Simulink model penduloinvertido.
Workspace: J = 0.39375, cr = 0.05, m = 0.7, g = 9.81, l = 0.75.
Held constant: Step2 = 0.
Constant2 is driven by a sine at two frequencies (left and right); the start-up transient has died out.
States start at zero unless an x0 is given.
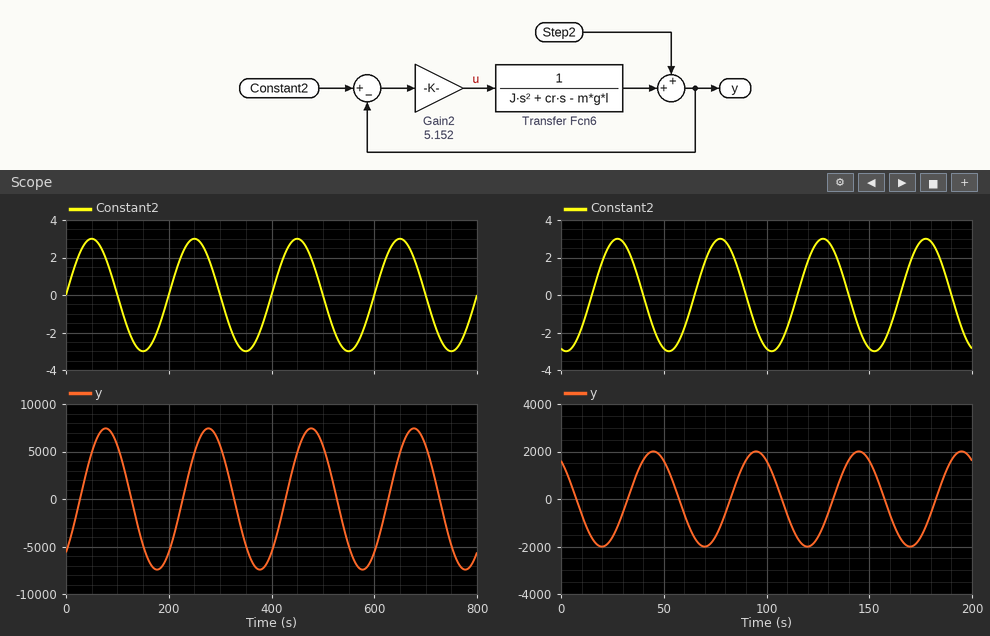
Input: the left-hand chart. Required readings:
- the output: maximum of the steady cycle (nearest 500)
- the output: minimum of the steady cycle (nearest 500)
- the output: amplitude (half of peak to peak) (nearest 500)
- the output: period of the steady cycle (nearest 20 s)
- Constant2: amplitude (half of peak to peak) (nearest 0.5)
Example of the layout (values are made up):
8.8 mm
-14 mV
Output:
7500
-7500
7500
200 s
3.0
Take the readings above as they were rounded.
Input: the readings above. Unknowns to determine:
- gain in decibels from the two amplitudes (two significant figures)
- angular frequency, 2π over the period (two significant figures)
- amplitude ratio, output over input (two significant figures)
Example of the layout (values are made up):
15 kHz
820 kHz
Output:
68 dB
0.031 rad/s
2500
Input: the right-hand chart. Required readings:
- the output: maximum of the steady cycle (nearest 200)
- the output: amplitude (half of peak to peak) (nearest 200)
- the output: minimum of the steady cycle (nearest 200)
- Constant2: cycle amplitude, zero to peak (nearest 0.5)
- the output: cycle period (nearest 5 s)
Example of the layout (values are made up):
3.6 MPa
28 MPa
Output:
2000
2000
-2000
3.0
50 s
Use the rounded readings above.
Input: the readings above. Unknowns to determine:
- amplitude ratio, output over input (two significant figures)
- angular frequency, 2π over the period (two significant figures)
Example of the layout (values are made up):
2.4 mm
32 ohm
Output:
670
0.13 rad/s
